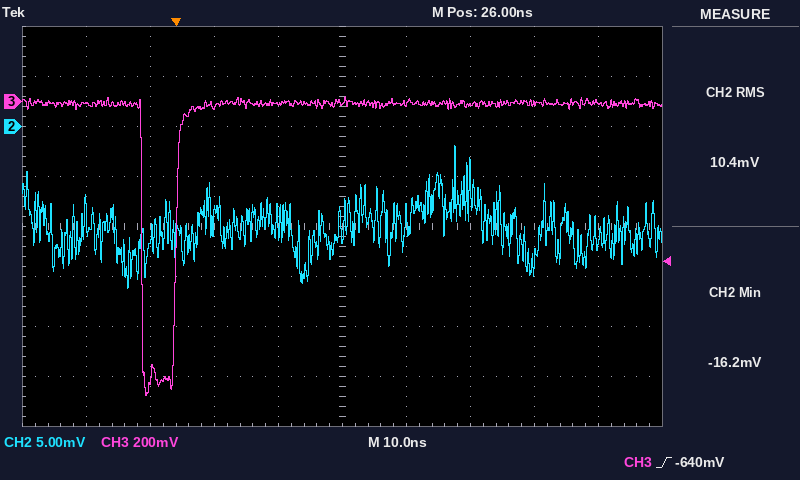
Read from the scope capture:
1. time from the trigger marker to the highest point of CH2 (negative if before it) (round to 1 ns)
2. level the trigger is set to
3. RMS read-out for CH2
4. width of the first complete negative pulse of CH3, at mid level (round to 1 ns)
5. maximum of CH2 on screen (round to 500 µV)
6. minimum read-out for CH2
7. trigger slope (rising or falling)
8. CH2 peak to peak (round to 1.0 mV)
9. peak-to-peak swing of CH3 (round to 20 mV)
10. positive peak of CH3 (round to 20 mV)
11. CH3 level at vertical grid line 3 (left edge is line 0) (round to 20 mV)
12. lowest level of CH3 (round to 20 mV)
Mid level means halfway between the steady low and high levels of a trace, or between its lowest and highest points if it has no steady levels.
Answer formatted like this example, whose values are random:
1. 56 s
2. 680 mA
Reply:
1. +44 ns
2. -640 mV
3. 10.4 mV
4. 5 ns
5. -2.0 mV
6. -16.2 mV
7. rising
8. 14.0 mV
9. 1.20 V
10. 20 mV
11. -20 mV
12. -1.18 V
